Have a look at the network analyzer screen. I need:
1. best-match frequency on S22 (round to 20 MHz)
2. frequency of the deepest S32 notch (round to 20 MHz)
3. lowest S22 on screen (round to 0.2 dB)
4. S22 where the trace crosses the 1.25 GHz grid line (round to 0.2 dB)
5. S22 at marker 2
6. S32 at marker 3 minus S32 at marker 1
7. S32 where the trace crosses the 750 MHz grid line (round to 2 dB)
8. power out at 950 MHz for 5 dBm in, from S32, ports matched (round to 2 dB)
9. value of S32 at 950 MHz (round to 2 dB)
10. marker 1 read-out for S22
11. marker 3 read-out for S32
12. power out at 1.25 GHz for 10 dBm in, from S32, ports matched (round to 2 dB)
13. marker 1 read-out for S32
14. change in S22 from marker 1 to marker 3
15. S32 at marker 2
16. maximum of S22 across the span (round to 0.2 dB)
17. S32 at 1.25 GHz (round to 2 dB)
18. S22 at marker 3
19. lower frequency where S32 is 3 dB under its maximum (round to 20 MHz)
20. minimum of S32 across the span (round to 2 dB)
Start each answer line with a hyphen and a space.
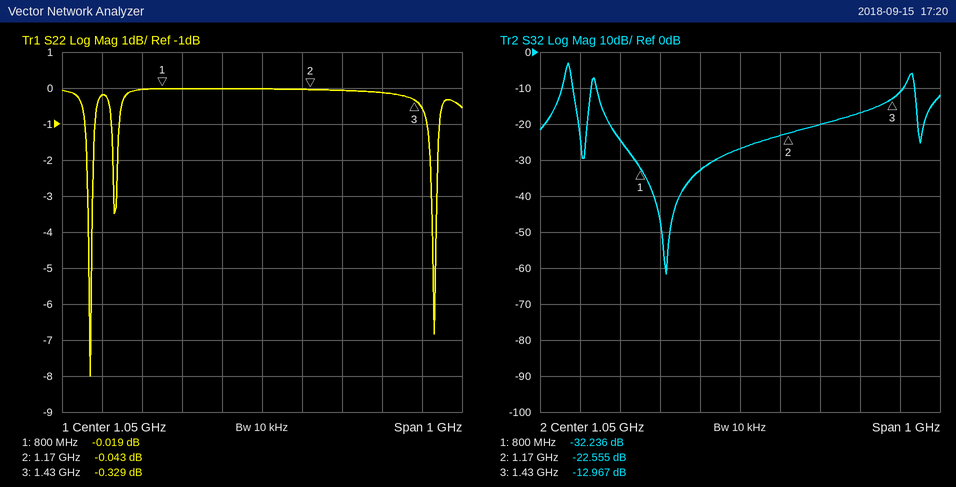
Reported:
- 620 MHz
- 860 MHz
- -8.0 dB
- 0.0 dB
- -0.043 dB
- 19.269 dB
- -24 dB
- -28 dBm
- -32 dB
- -0.019 dB
- -12.967 dB
- -10 dBm
- -32.236 dB
- -0.310 dB
- -22.555 dB
- 0.0 dB
- -20 dB
- -0.329 dB
- 620 MHz
- -62 dB
